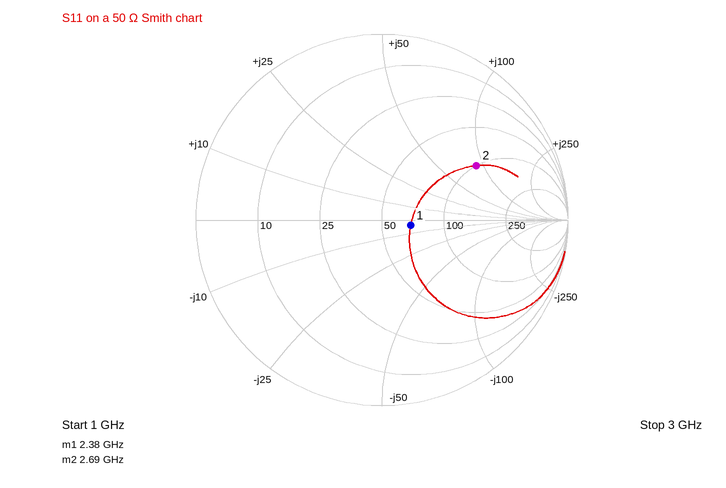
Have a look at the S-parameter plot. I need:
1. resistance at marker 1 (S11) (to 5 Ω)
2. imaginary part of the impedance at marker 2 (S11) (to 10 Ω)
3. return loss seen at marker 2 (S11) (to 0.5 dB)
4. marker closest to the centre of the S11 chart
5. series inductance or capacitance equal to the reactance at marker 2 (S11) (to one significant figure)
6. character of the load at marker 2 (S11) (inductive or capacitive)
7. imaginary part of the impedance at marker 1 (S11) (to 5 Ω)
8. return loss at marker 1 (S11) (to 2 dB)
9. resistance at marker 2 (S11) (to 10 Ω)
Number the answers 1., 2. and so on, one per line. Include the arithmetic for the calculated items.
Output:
1. 70 Ω
2. +90 Ω
3. 4.5 dB
4. marker 1
5. L = 90 Ω/(2π × 2.69 GHz) ≈ 5 nH
6. inductive
7. -5 Ω
8. 16 dB
9. 100 Ω
